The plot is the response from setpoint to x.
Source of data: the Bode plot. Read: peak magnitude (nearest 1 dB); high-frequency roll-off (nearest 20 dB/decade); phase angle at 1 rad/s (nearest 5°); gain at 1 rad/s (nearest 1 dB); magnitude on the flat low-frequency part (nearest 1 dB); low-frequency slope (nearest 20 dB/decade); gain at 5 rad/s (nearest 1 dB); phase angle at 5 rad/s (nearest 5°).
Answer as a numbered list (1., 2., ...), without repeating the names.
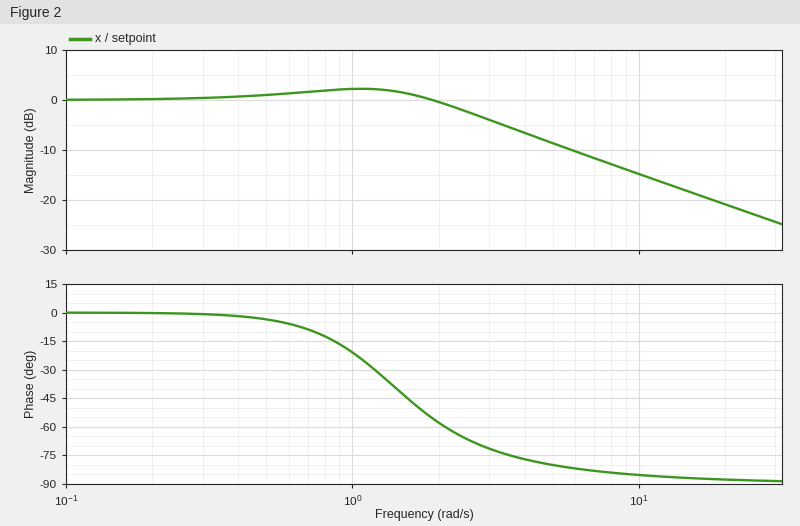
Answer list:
1. 2 dB
2. -20 dB/decade
3. -20°
4. 2 dB
5. 0 dB
6. 0 dB/decade
7. -9 dB
8. -80°
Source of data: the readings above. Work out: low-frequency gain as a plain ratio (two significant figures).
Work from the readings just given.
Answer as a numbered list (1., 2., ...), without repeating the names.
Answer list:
1. 1.0
